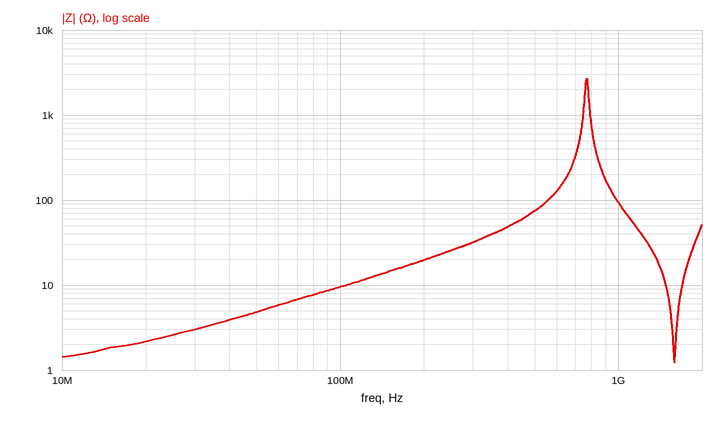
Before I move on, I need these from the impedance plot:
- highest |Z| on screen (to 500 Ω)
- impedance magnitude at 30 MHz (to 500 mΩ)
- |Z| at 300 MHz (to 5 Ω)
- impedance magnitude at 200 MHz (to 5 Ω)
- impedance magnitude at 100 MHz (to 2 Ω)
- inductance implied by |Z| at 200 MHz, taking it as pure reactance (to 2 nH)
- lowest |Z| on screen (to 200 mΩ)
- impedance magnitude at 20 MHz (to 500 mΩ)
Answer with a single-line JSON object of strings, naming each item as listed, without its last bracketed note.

{"highest |Z| on screen": "2.5 kΩ", "impedance magnitude at 30 MHz": "3.0 Ω", "|Z| at 300 MHz": "30 Ω", "impedance magnitude at 200 MHz": "20 Ω", "impedance magnitude at 100 MHz": "10 Ω", "inductance implied by |Z| at 200 MHz, taking it as pure reactance": "16 nH", "lowest |Z| on screen": "1.2 Ω", "impedance magnitude at 20 MHz": "2.0 Ω"}
